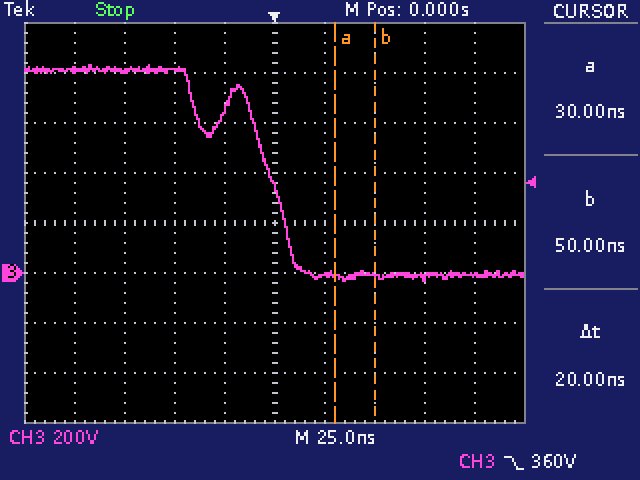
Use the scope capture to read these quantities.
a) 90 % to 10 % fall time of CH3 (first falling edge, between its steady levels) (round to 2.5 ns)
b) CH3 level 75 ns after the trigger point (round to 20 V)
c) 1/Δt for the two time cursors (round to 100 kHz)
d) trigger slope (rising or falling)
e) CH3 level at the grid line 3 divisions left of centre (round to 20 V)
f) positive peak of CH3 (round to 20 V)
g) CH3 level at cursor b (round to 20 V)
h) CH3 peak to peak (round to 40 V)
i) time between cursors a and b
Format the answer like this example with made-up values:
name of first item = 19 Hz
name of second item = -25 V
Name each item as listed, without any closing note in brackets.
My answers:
90 % to 10 % fall time of CH3 (first falling edge, between its steady levels) = 25.0 ns
CH3 level 75 ns after the trigger point = -20 V
1/Δt for the two time cursors = 50.0 MHz
trigger slope = falling
CH3 level at the grid line 3 divisions left of centre = 800 V
positive peak of CH3 = 840 V
CH3 level at cursor b = -20 V
CH3 peak to peak = 880 V
time between cursors a and b = 20 ns
